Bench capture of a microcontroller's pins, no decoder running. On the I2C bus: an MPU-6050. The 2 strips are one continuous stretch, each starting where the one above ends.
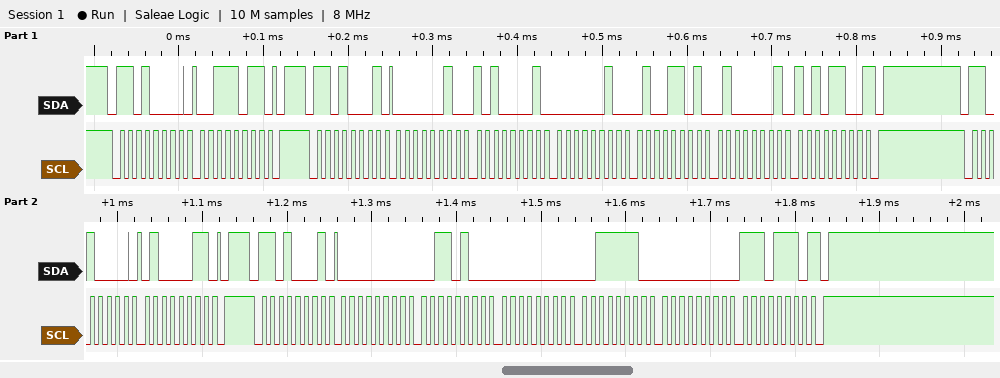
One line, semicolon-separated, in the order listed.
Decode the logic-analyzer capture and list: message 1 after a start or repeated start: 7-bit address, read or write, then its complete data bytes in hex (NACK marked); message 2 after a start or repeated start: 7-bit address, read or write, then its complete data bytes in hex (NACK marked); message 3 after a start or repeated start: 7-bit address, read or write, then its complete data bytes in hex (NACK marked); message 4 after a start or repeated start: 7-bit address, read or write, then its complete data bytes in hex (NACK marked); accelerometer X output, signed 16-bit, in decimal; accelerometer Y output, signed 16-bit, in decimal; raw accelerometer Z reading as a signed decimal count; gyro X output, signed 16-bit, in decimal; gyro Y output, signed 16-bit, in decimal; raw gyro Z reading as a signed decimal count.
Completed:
0x68 write: 3B; 0x68 read: 02 A1 02 4D 41 AC NACK; 0x68 write: 43; 0x68 read: 00 34 00 3E 00 EE NACK; 673; 589; 16812; 52; 62; 238
